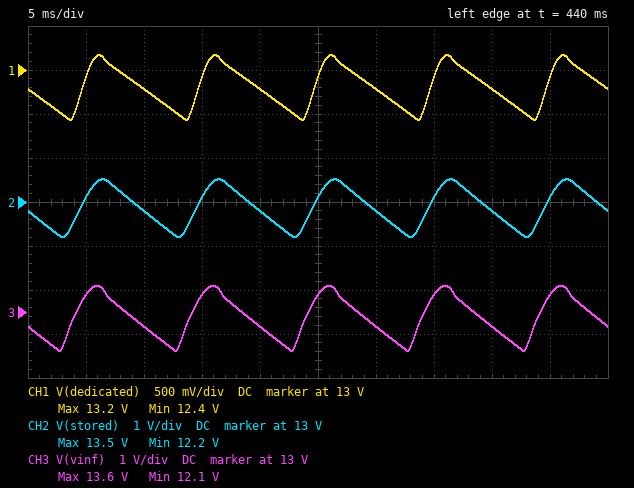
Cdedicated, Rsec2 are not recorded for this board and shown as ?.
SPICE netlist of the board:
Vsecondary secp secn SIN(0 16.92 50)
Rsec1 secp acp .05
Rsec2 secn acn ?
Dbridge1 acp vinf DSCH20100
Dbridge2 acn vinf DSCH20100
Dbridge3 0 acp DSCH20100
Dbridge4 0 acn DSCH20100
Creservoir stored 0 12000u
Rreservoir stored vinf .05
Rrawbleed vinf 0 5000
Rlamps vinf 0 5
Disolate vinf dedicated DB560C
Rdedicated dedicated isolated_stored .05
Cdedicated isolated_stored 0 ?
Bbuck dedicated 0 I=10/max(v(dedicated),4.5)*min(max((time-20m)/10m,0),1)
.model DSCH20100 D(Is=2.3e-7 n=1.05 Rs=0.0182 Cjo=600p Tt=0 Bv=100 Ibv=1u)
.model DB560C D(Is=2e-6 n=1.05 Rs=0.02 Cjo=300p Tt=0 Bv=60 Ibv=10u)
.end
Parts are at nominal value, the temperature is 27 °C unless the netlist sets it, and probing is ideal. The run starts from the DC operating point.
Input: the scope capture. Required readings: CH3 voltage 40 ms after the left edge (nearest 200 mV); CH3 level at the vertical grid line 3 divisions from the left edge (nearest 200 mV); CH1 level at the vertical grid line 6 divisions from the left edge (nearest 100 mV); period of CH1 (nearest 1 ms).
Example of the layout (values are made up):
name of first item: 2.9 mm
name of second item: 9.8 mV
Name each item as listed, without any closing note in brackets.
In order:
CH3 voltage 40 ms after the left edge: 12.6 V
CH3 level at the vertical grid line 3 divisions from the left edge: 13.4 V
CH1 level at the vertical grid line 6 divisions from the left edge: 12.8 V
period of CH1: 10 ms
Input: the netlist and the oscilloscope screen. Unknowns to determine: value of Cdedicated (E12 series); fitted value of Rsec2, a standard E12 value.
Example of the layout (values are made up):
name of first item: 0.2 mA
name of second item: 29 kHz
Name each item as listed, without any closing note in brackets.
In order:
value of Cdedicated: 8.2 mF
fitted value of Rsec2, a standard E12 value: 0.12 Ω
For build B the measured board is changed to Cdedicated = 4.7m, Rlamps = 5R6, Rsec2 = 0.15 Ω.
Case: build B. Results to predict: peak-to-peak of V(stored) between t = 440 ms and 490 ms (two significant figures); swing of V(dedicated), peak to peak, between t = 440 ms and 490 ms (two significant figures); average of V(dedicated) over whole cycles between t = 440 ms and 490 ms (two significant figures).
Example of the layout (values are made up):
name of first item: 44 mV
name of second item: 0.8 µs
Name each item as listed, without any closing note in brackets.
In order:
peak-to-peak of V(stored) between t = 440 ms and 490 ms: 1.2 V
swing of V(dedicated), peak to peak, between t = 440 ms and 490 ms: 1.1 V
average of V(dedicated) over whole cycles between t = 440 ms and 490 ms: 13 V
